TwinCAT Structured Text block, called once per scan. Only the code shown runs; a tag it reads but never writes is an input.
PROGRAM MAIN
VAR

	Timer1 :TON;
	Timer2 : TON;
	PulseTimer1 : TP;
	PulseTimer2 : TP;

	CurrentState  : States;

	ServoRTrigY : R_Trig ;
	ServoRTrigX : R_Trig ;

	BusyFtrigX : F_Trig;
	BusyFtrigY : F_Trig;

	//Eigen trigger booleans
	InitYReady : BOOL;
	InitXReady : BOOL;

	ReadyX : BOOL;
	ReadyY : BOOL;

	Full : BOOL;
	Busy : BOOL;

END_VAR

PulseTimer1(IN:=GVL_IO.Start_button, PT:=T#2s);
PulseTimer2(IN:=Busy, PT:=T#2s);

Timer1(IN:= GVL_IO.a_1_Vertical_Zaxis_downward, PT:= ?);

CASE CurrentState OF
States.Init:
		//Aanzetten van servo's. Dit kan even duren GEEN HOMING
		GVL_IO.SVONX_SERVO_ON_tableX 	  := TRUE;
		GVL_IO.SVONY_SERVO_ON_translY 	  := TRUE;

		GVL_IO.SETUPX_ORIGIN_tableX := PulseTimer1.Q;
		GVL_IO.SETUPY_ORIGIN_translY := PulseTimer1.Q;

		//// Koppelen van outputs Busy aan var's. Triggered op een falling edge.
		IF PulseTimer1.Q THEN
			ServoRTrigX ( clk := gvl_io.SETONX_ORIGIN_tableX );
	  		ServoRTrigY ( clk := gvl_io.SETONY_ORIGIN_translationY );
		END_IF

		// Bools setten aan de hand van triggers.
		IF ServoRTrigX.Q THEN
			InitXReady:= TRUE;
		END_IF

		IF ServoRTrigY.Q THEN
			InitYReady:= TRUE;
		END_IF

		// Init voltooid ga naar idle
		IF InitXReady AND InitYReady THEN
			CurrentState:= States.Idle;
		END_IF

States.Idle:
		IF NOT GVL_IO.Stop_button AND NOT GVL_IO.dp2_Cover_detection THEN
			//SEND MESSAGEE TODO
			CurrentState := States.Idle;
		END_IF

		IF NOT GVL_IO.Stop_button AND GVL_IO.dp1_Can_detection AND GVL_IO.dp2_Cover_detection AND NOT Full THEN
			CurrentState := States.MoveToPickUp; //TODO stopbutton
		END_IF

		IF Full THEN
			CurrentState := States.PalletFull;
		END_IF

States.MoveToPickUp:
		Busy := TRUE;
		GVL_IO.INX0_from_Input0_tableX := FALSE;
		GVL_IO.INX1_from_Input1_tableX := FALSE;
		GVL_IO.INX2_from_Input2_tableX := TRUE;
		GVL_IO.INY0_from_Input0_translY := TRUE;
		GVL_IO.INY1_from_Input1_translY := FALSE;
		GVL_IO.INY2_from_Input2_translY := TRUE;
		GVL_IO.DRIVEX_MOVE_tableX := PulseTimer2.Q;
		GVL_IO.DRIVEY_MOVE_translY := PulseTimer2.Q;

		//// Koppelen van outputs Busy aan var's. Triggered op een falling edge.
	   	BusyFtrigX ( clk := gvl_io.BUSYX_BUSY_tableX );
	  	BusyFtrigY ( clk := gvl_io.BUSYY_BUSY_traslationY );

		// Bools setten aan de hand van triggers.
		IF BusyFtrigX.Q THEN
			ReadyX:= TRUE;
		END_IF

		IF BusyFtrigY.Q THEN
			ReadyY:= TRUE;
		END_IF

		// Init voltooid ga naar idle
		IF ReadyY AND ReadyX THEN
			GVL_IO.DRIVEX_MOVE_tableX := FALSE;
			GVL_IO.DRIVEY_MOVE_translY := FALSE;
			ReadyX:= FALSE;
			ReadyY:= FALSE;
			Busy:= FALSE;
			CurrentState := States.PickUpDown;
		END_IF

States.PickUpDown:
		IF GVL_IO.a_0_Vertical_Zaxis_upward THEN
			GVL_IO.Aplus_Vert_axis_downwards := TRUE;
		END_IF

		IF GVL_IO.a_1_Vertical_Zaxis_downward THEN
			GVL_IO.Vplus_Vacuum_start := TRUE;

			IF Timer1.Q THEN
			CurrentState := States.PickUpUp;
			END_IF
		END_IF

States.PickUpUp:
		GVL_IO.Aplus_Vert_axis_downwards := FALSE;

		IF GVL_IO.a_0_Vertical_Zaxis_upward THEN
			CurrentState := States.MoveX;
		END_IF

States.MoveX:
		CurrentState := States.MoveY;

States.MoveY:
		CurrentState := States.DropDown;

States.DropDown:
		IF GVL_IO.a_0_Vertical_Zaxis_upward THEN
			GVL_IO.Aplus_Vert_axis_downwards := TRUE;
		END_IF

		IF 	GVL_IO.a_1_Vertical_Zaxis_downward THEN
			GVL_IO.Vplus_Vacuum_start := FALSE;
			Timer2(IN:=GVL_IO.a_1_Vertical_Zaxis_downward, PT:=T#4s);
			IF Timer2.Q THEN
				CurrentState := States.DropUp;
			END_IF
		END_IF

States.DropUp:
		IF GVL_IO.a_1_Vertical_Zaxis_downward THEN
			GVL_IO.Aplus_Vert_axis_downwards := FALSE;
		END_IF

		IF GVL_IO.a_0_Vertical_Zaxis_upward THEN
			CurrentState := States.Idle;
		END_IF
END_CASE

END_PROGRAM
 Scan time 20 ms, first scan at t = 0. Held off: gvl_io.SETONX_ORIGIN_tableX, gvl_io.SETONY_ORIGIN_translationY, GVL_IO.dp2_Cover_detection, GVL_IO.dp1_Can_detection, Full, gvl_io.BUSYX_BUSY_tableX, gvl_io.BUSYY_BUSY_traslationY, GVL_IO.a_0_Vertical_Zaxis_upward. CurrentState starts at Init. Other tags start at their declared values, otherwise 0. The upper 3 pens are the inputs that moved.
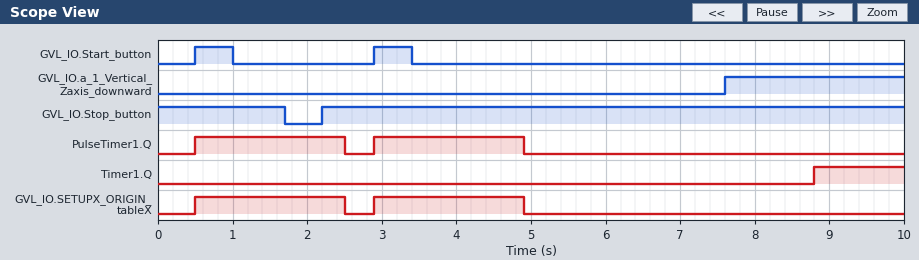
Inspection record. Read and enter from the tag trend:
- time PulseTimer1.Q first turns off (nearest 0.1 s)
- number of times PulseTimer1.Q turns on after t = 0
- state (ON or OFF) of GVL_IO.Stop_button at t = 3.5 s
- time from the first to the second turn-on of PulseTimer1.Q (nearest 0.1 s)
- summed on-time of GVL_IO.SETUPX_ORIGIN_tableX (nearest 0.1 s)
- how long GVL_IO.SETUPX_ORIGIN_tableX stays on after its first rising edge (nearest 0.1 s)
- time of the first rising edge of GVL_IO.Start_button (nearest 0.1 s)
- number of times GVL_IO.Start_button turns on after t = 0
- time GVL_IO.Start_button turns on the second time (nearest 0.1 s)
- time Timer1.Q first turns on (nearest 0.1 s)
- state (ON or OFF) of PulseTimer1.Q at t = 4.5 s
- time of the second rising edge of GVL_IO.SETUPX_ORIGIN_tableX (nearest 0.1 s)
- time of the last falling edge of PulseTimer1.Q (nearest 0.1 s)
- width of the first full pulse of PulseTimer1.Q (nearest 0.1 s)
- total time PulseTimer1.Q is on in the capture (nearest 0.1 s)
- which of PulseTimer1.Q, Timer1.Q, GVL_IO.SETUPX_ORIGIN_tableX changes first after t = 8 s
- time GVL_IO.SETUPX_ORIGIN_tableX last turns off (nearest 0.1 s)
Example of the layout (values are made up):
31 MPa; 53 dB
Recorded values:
2.5 s; 2; ON; 2.4 s; 4.0 s; 2.0 s; 0.5 s; 2; 2.9 s; 8.8 s; ON; 2.9 s; 4.9 s; 2.0 s; 4.0 s; Timer1.Q; 4.9 s
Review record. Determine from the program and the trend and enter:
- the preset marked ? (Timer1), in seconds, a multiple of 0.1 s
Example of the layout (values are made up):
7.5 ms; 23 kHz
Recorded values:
1.2 s
